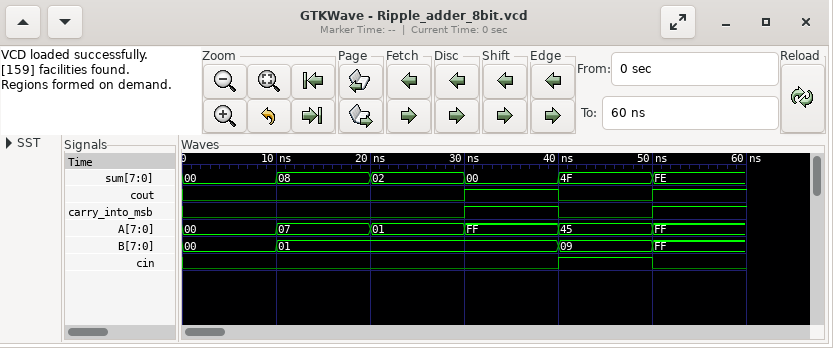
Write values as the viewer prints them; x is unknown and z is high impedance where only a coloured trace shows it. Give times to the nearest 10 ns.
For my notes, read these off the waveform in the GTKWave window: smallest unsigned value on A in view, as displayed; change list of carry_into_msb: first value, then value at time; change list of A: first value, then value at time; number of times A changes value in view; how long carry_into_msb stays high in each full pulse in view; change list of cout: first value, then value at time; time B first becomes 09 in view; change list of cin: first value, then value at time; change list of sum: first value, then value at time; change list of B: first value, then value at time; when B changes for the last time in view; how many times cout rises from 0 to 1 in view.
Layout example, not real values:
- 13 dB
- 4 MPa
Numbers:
- 00
- 0, 1 at 30 ns, 0 at 40 ns, 1 at 50 ns
- 00, 07 at 10 ns, 01 at 20 ns, FF at 30 ns, 45 at 40 ns, FF at 50 ns
- 5
- 10 ns
- 0, 1 at 30 ns, 0 at 40 ns, 1 at 50 ns
- 40 ns
- 0, 1 at 40 ns, 0 at 50 ns
- 00, 08 at 10 ns, 02 at 20 ns, 00 at 30 ns, 4F at 40 ns, FE at 50 ns
- 00, 01 at 10 ns, 09 at 40 ns, FF at 50 ns
- 50 ns
- 2
